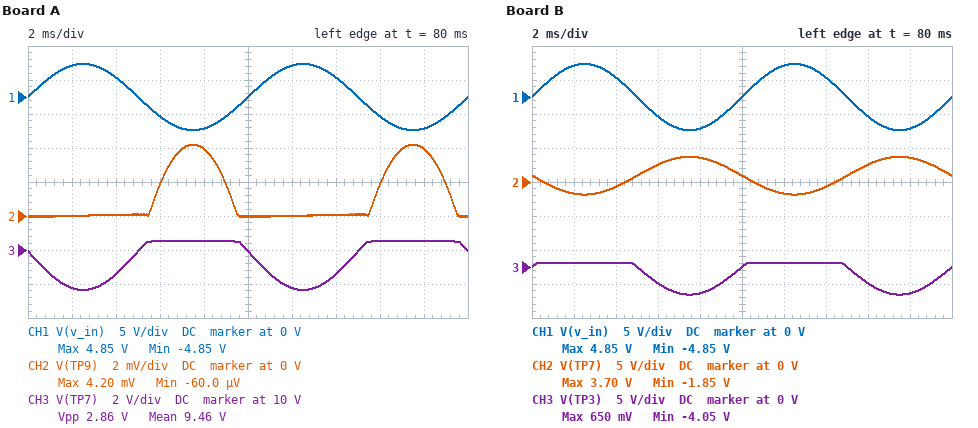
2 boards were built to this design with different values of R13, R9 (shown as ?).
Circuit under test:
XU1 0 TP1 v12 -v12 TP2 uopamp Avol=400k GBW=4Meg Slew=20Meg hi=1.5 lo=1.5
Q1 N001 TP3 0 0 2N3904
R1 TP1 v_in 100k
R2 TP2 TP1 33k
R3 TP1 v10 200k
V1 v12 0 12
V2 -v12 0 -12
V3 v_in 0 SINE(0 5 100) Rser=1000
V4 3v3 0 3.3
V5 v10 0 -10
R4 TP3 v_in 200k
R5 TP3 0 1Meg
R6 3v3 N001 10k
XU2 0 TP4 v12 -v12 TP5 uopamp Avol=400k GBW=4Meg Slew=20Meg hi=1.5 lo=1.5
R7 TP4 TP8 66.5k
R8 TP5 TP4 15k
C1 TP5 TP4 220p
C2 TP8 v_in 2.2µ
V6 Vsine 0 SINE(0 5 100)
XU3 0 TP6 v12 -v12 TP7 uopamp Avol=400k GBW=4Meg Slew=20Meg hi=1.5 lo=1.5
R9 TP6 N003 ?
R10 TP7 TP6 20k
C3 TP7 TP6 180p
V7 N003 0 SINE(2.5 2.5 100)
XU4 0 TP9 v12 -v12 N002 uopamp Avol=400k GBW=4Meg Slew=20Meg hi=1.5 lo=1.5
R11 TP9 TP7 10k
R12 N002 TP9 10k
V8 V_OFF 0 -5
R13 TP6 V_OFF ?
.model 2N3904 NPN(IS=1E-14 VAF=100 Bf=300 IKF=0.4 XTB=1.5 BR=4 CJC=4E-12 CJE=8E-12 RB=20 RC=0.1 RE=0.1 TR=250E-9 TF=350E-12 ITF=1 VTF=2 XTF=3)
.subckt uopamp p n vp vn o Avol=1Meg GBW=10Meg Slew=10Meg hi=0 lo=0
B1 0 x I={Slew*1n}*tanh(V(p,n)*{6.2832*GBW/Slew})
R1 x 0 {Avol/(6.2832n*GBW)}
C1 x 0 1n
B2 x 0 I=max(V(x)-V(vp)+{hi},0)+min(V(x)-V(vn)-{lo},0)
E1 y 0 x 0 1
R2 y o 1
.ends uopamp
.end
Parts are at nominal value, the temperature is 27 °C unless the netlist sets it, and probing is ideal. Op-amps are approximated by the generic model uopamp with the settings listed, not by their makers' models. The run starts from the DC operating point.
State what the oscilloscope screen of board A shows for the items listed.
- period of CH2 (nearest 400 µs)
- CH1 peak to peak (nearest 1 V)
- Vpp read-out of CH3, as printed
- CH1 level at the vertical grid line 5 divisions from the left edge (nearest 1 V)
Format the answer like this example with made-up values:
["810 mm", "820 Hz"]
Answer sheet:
["10.0 ms", "10 V", "2.86 V", "0 V"]
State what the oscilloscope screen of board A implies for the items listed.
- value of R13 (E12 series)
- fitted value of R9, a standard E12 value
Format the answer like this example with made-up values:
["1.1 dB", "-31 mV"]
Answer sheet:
["8.2 kΩ", "22 kΩ"]
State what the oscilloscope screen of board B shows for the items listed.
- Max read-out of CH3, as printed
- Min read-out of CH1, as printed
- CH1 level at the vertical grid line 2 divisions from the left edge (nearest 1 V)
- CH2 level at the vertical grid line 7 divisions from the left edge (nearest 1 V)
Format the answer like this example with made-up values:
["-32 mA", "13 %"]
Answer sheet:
["650 mV", "-4.85 V", "3 V", "-1 V"]
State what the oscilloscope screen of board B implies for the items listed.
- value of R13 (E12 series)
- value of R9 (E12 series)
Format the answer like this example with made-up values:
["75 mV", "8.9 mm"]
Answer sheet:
["27 kΩ", "18 kΩ"]
